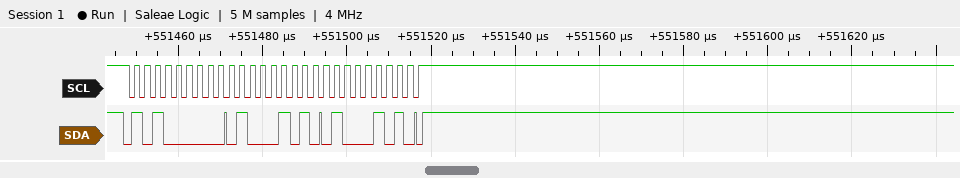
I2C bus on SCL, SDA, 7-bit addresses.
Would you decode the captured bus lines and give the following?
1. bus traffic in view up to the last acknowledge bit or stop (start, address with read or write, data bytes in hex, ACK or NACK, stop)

start, address 50 write ACK, 45 ACK, 45 ACK, stop
